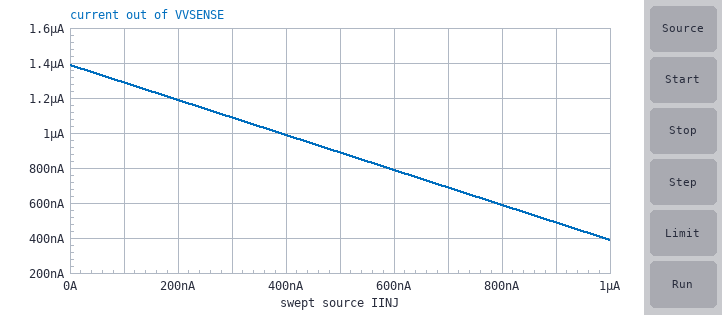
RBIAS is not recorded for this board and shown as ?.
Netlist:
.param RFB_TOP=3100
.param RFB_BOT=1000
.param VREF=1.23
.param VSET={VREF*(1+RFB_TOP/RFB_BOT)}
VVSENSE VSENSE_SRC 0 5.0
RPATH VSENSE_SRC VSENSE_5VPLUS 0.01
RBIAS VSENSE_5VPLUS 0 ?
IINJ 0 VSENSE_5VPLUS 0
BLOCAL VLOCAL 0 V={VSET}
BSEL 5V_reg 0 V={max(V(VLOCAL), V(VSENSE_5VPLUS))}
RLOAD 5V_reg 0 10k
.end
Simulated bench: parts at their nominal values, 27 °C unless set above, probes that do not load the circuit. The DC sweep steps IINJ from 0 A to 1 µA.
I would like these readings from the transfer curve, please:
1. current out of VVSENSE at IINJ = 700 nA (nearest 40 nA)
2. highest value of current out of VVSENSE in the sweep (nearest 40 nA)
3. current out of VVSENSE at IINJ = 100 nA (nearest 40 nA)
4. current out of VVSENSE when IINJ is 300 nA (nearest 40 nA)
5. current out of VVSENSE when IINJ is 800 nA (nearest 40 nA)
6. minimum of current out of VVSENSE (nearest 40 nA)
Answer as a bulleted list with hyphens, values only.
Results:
- 680 nA
- 1.40 µA
- 1.28 µA
- 1.08 µA
- 600 nA
- 400 nA
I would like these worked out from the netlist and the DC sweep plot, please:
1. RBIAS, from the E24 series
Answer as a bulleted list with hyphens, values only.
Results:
- 3.6 MΩ
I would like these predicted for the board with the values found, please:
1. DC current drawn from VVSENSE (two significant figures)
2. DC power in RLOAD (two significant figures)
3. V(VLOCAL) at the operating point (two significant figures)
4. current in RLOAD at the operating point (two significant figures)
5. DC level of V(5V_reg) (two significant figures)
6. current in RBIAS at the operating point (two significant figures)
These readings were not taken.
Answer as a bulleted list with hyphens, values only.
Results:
- 1.4 µA
- 2.5 mW
- 5.0 V
- 500 µA
- 5.0 V
- 1.4 µA
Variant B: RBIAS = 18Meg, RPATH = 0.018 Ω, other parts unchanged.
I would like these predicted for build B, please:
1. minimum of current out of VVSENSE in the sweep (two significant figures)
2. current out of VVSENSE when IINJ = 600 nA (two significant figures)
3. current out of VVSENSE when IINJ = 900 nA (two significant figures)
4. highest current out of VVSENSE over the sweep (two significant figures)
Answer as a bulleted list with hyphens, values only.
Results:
- -720 nA
- -320 nA
- -620 nA
- 280 nA
